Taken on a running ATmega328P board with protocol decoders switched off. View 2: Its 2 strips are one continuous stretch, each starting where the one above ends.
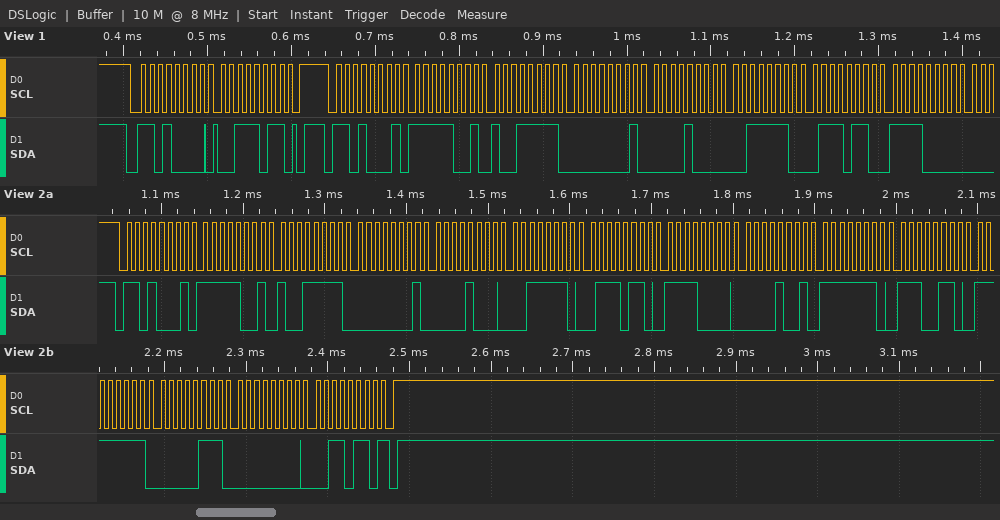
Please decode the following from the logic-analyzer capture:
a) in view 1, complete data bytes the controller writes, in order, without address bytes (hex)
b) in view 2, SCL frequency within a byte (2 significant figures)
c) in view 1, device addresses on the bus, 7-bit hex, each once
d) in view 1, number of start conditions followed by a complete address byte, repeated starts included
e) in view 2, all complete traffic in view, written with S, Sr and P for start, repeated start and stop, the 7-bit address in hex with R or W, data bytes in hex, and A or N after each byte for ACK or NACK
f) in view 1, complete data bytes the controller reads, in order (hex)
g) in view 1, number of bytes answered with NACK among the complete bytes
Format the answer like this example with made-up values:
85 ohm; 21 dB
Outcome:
3B; 100 kHz; 0x68; 2; S 68R A F9 A 9F A 01 A 08 A 3E A 76 A F0 A 09 A FE A E6 A FF A 07 A 00 A 36 N P; F9 9F 01 08 3E 76 F0; 0
